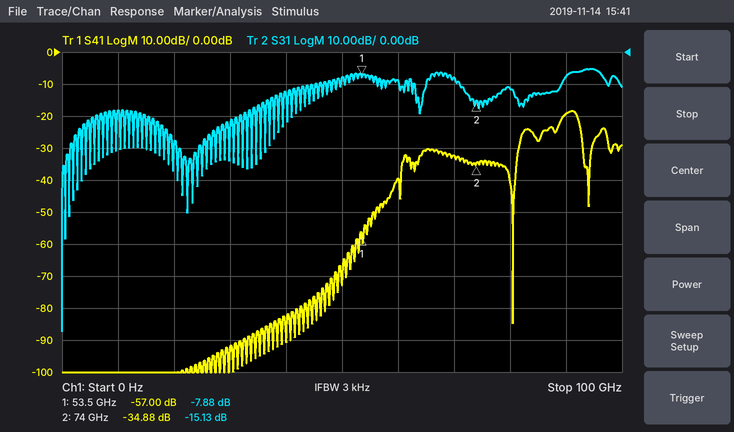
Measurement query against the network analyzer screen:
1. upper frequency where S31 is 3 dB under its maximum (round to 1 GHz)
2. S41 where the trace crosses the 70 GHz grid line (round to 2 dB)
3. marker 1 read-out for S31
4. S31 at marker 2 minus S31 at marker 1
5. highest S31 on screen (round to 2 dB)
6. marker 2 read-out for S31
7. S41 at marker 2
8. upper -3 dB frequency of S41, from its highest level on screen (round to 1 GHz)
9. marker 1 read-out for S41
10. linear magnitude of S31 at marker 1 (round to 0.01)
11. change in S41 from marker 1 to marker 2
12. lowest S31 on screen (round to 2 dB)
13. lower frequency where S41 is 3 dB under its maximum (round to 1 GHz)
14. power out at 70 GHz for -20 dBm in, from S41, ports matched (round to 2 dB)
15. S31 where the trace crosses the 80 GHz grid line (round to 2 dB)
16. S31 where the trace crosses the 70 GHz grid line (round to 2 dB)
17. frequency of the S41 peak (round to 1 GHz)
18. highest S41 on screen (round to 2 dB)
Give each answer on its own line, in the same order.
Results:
97 GHz
-32 dB
-7.88 dB
-7.25 dB
-6 dB
-15.13 dB
-34.88 dB
92 GHz
-57.00 dB
0.40
22.12 dB
-88 dB
89 GHz
-52 dBm
-12 dB
-8 dB
91 GHz
-18 dB
